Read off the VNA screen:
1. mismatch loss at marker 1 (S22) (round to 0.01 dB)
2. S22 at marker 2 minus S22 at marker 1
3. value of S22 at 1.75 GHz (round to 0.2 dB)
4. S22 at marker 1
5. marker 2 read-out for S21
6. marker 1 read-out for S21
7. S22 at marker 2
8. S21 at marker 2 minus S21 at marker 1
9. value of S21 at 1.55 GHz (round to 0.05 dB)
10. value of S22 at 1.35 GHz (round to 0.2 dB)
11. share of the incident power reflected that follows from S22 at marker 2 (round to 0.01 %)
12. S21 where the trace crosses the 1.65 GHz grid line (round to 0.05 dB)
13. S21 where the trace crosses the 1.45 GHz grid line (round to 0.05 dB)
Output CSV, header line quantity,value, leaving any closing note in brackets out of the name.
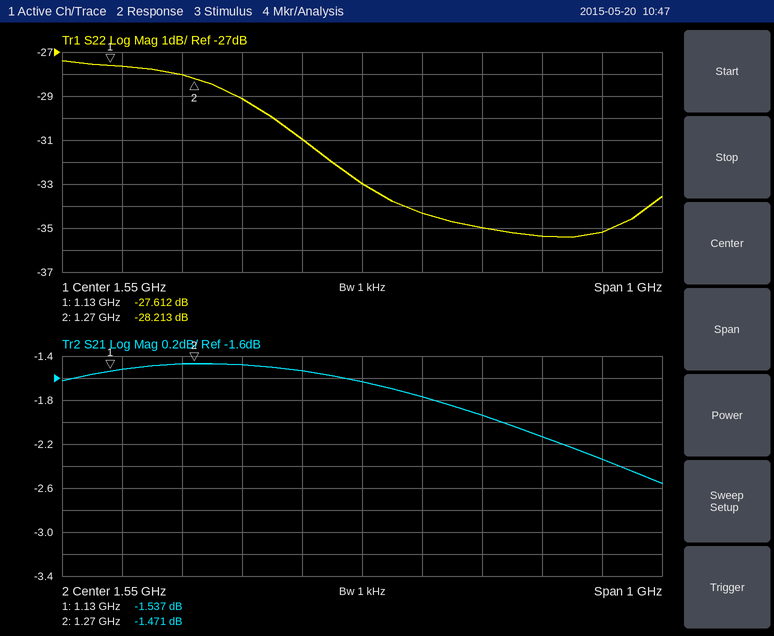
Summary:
quantity,value
mismatch loss at marker 1 (S22),0.01 dB
S22 at marker 2 minus S22 at marker 1,-0.601 dB
value of S22 at 1.75 GHz,-35.0 dB
S22 at marker 1,-27.612 dB
marker 2 read-out for S21,-1.471 dB
marker 1 read-out for S21,-1.537 dB
S22 at marker 2,-28.213 dB
S21 at marker 2 minus S21 at marker 1,0.066 dB
value of S21 at 1.55 GHz,-1.65 dB
value of S22 at 1.35 GHz,-29.2 dB
share of the incident power reflected that follows from S22 at marker 2,0.15 %
S21 where the trace crosses the 1.65 GHz grid line,-1.75 dB
S21 where the trace crosses the 1.45 GHz grid line,-1.55 dB
